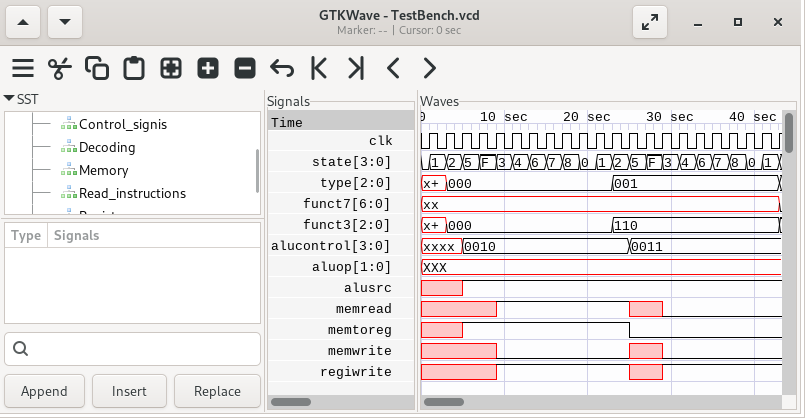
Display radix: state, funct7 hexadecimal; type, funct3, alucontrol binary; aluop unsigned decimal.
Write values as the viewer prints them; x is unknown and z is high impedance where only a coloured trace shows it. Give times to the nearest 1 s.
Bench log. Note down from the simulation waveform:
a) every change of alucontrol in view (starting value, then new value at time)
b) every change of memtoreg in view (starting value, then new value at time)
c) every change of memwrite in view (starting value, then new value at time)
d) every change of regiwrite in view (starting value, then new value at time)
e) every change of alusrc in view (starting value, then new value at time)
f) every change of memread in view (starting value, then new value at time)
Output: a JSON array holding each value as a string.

["xxxx, 0010 at 5 s, 0011 at 25 s", "x, 1 at 5 s, 0 at 25 s", "x, 0 at 9 s, x at 25 s, 0 at 29 s", "x, 1 at 9 s, x at 25 s, 1 at 29 s", "x, 1 at 5 s", "x, 1 at 9 s, x at 25 s, 0 at 29 s"]
